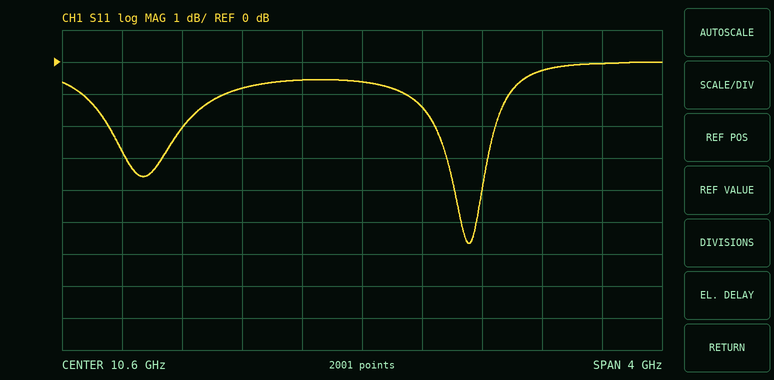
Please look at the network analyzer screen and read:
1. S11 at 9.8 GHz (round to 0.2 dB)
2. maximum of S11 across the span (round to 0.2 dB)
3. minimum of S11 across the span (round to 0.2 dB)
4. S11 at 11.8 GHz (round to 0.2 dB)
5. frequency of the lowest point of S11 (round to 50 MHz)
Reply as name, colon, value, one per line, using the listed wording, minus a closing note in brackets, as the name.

S11 at 9.8 GHz: -0.8 dB
maximum of S11 across the span: 0.0 dB
minimum of S11 across the span: -5.6 dB
S11 at 11.8 GHz: -0.2 dB
frequency of the lowest point of S11: 11.30 GHz
